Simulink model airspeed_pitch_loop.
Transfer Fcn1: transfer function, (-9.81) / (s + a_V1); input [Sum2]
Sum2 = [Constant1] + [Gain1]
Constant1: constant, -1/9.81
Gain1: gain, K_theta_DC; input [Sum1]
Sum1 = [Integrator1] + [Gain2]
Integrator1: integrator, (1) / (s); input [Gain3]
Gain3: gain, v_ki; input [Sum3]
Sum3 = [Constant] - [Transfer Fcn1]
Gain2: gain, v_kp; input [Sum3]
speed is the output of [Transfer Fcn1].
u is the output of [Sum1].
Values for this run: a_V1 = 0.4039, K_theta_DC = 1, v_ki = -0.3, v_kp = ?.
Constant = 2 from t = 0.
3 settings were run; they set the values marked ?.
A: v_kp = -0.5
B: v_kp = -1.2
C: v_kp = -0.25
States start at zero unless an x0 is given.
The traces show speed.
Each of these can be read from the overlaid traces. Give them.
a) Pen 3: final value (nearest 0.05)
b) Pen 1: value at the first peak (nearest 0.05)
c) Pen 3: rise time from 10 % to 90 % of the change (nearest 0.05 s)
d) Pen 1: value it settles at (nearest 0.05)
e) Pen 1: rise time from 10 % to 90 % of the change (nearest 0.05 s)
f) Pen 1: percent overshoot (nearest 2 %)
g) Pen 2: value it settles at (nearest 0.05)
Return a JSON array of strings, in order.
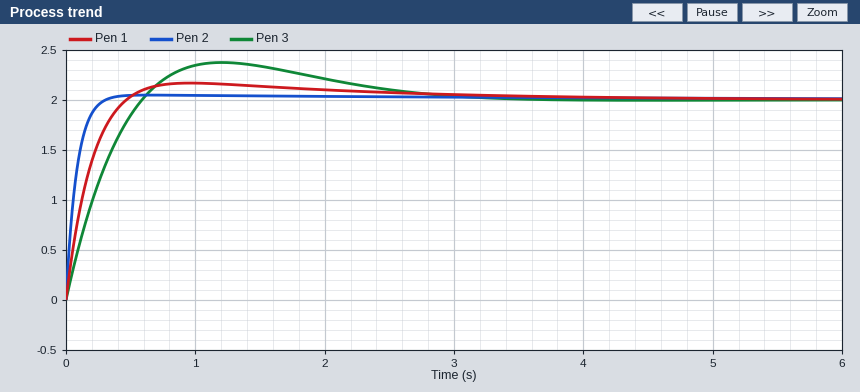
["2.00", "2.15", "0.45 s", "2.00", "0.30 s", "8 %", "2.00"]
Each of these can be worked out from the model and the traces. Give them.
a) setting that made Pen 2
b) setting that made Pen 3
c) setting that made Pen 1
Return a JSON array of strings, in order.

["B", "C", "A"]
